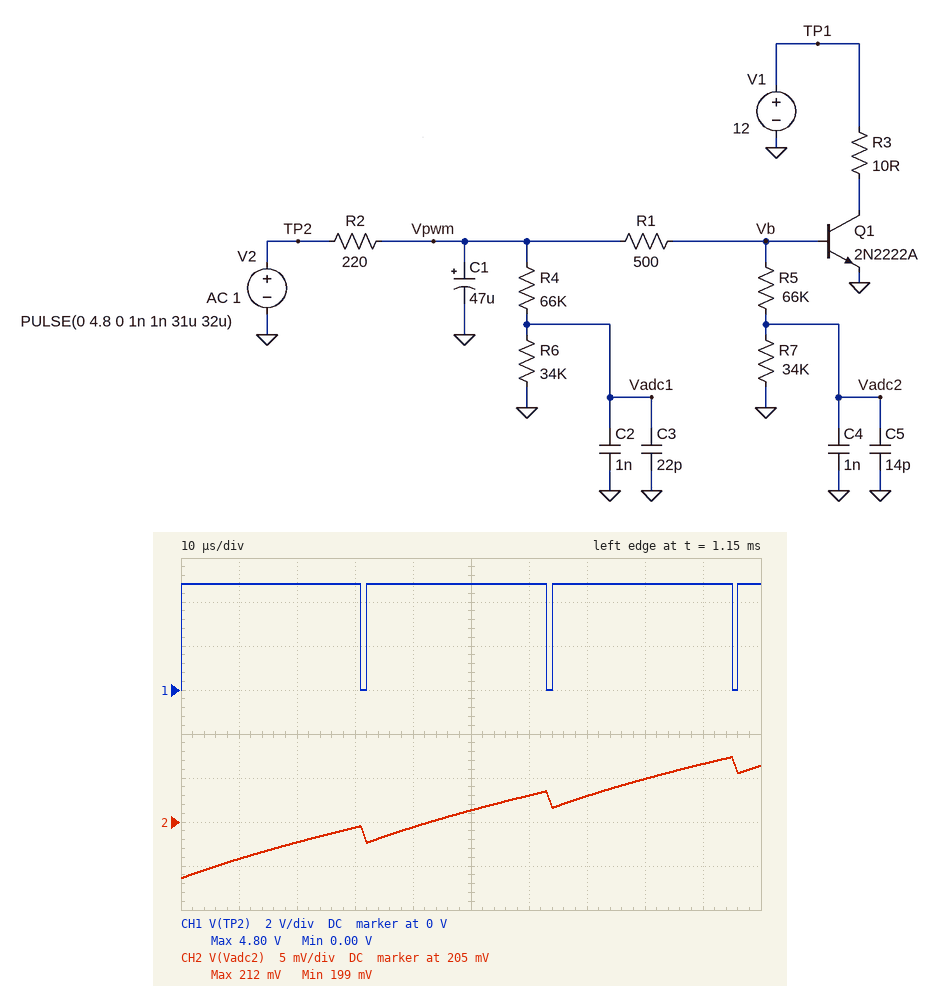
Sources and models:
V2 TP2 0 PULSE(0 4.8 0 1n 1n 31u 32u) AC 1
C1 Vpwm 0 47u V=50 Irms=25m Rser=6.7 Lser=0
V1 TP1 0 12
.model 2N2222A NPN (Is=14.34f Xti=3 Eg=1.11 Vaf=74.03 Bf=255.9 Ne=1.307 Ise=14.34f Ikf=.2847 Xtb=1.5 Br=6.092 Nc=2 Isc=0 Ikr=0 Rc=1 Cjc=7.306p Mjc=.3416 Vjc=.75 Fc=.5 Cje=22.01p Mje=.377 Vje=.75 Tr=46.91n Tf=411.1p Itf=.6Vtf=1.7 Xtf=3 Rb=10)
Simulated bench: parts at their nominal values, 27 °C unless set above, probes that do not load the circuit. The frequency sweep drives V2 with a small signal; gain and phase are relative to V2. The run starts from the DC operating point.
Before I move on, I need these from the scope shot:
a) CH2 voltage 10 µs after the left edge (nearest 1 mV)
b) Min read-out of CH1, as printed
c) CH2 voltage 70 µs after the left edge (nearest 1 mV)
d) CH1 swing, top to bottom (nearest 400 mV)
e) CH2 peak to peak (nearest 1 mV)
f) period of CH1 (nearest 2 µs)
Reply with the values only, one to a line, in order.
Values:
201 mV
0.00 V
208 mV
4.8 V
14 mV
32 µs
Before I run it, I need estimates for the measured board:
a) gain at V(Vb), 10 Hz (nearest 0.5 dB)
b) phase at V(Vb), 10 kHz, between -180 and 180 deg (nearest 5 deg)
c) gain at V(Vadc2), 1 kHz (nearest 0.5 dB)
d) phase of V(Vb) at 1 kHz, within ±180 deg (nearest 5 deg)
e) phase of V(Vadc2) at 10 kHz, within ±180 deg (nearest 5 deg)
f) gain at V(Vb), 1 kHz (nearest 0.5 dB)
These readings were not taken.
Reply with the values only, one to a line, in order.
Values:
-1.5 dB
-5 deg
-39.0 dB
-25 deg
-60 deg
-29.5 dB
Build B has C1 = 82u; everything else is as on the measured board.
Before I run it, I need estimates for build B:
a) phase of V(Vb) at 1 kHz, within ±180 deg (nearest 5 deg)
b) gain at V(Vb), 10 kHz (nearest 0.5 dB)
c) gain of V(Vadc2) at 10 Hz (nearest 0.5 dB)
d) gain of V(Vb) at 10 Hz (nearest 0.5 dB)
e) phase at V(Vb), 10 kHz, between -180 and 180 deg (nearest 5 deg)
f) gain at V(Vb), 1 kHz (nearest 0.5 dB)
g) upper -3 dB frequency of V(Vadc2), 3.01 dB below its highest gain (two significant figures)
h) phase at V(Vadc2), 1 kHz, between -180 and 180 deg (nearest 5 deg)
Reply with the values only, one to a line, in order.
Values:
-15 deg
-30.5 dB
-13.0 dB
-4.0 dB
0 deg
-30.5 dB
8.6 Hz
-25 deg
